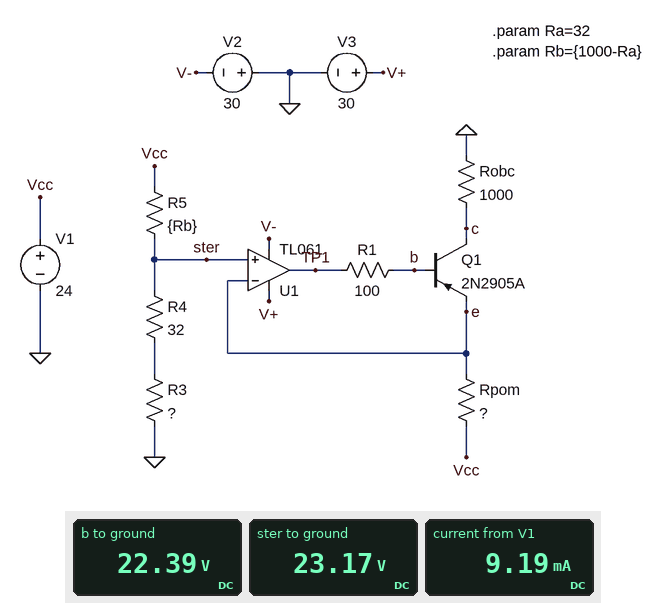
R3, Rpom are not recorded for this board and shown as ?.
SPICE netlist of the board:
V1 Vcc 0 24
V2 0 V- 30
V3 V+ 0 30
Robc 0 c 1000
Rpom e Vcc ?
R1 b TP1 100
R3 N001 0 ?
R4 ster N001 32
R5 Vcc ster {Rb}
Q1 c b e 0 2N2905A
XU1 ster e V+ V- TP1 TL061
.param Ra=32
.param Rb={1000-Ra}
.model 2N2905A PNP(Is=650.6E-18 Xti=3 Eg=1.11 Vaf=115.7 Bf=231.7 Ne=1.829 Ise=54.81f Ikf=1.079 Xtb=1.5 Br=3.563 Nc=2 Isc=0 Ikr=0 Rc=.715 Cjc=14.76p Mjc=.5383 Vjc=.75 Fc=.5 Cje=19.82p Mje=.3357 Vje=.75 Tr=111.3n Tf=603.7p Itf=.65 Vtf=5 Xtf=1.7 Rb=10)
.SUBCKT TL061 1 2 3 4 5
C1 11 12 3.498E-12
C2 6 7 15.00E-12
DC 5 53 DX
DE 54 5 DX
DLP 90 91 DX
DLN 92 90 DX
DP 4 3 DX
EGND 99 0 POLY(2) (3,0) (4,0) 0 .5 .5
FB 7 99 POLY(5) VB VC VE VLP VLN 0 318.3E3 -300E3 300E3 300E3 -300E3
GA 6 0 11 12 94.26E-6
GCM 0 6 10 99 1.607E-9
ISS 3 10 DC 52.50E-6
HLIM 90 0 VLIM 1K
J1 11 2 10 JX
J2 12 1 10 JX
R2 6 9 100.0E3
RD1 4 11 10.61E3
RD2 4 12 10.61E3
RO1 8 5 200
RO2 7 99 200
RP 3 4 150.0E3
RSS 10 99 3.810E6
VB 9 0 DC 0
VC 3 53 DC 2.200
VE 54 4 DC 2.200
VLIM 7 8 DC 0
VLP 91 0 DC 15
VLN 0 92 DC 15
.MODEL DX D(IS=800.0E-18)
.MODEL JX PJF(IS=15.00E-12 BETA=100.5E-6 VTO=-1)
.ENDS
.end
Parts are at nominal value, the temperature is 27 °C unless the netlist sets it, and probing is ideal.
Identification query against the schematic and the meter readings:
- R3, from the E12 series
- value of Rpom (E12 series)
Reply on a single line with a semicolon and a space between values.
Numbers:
27 kΩ; 100 Ω
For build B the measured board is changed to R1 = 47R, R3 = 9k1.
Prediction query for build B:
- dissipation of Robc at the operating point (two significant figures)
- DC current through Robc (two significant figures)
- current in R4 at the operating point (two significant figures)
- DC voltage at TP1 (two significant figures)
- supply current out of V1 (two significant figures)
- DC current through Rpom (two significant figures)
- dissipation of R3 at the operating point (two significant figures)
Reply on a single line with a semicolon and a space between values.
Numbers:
470 mW; 22 mA; 2.4 mA; 21 V; 25 mA; 23 mA; 51 mW
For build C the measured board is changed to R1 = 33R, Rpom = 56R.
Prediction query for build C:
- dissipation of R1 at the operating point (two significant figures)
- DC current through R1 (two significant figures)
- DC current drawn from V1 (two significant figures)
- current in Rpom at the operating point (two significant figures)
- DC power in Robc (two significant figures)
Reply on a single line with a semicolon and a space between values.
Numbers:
130 nW; 62 µA; 16 mA; 15 mA; 220 mW
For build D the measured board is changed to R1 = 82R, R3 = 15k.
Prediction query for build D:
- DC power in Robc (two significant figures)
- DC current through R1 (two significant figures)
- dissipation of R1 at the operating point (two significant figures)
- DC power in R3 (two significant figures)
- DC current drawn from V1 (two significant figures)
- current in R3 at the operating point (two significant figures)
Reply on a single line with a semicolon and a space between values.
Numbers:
210 mW; 61 µA; 300 nW; 34 mW; 16 mA; 1.5 mA
